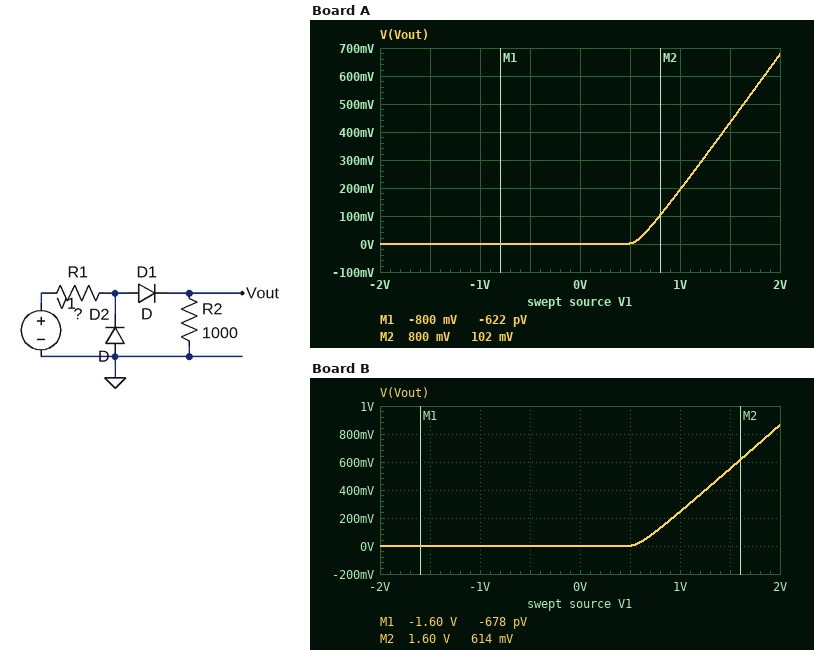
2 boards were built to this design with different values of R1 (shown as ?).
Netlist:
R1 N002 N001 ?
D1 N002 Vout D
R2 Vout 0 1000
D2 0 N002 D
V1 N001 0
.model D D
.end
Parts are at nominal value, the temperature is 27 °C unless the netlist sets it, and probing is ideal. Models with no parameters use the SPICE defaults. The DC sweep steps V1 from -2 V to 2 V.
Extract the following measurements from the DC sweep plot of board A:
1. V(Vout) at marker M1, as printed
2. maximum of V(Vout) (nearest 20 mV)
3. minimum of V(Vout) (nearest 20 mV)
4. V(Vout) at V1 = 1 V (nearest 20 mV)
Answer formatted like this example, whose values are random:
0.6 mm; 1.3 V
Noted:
-622 pV; 680 mV; 0 V; 200 mV
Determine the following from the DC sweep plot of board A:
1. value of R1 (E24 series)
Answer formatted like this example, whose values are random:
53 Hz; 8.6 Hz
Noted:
1 kΩ
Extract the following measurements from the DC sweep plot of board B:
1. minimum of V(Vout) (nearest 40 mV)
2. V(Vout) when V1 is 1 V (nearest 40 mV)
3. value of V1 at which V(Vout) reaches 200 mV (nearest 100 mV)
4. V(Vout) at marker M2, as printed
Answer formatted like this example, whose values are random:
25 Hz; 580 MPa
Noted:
0 V; 240 mV; 900 mV; 614 mV
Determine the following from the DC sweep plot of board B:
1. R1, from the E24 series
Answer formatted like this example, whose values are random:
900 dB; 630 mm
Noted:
560 Ω
